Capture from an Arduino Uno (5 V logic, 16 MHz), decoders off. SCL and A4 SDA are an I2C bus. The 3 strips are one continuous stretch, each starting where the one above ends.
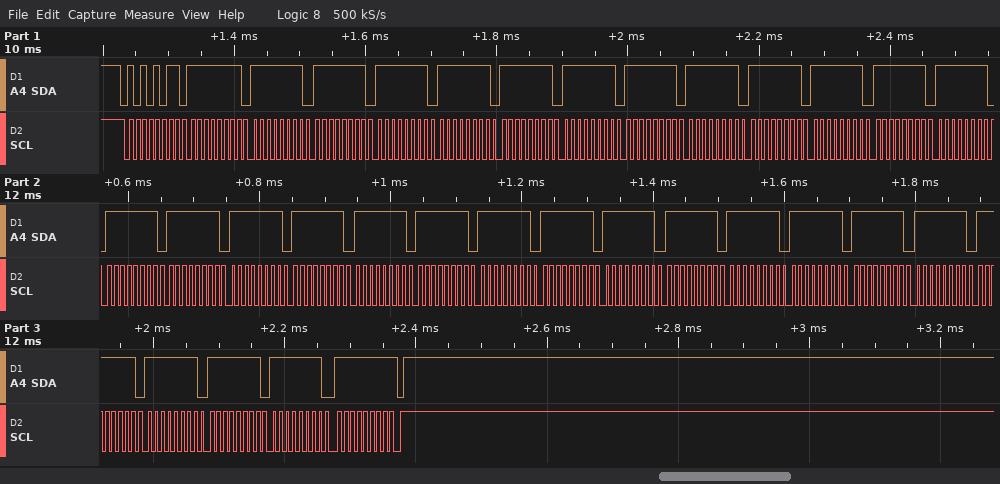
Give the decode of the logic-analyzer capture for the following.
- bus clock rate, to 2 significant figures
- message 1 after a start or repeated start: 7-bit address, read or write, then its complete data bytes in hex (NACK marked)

100 kHz
0x55 read: FF FF FF FF FF FF FF FF FF FF FF FF FF FF FF FF FF FF FF FF FF FF FF FF FF FF FF FF FF FF FF FF NACK
